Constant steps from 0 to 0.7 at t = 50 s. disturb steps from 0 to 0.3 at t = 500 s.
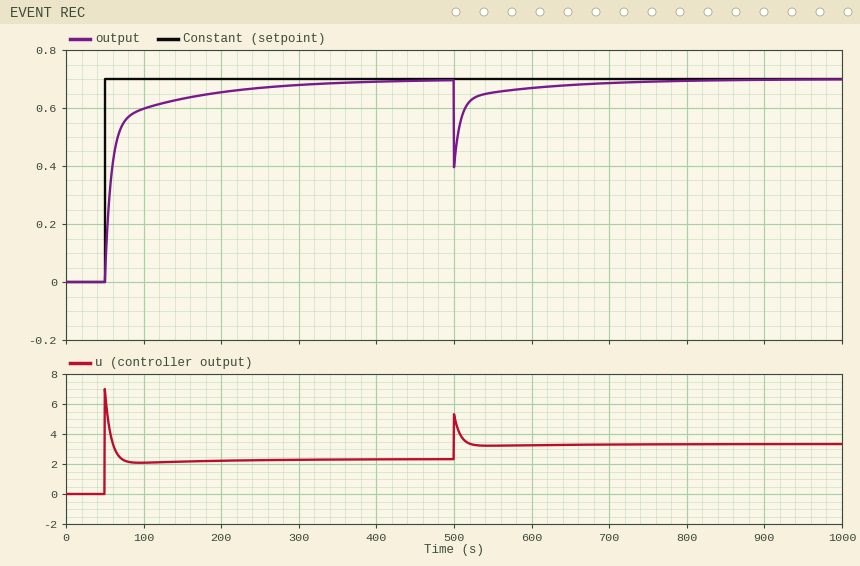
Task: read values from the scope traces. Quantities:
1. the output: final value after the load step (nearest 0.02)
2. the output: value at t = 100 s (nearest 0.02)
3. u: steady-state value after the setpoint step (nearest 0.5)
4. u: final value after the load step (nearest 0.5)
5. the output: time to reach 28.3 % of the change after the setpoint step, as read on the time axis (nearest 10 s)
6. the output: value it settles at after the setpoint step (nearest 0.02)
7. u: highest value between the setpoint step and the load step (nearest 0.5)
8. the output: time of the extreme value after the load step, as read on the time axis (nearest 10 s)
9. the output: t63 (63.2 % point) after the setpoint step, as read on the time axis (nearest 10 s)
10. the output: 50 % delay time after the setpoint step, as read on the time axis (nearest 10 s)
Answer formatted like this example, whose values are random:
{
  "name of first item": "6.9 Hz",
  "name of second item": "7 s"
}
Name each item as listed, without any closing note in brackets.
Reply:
{
  "the output: final value after the load step": "0.70",
  "the output: value at t = 100 s": "0.60",
  "u: steady-state value after the setpoint step": "2.5",
  "u: final value after the load step": "3.5",
  "the output: time to reach 28.3 % of the change after the setpoint step, as read on the time axis": "50 s",
  "the output: value it settles at after the setpoint step": "0.70",
  "u: highest value between the setpoint step and the load step": "7.0",
  "the output: time of the extreme value after the load step, as read on the time axis": "500 s",
  "the output: t63 (63.2 % point) after the setpoint step, as read on the time axis": "60 s",
  "the output: 50 % delay time after the setpoint step, as read on the time axis": "60 s"
}
